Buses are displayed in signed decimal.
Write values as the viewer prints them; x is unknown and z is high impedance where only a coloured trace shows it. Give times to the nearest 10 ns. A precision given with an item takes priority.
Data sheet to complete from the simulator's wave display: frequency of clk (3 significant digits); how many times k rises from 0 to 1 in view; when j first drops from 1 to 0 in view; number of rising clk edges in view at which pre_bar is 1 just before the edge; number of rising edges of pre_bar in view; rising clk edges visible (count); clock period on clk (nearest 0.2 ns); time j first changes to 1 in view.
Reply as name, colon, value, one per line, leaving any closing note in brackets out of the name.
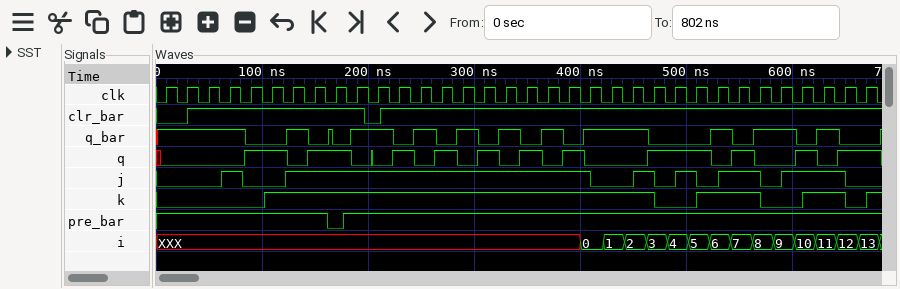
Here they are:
frequency of clk: 50.0 MHz
how many times k rises from 0 to 1 in view: 4
when j first drops from 1 to 0 in view: 80 ns
number of rising clk edges in view at which pre_bar is 1 just before the edge: 33
number of rising edges of pre_bar in view: 1
rising clk edges visible: 34
clock period on clk: 20 ns
time j first changes to 1 in view: 60 ns
